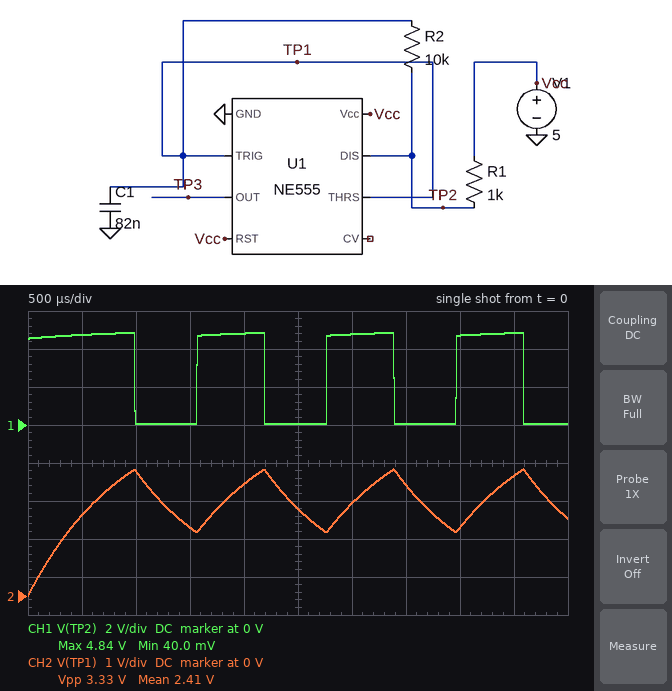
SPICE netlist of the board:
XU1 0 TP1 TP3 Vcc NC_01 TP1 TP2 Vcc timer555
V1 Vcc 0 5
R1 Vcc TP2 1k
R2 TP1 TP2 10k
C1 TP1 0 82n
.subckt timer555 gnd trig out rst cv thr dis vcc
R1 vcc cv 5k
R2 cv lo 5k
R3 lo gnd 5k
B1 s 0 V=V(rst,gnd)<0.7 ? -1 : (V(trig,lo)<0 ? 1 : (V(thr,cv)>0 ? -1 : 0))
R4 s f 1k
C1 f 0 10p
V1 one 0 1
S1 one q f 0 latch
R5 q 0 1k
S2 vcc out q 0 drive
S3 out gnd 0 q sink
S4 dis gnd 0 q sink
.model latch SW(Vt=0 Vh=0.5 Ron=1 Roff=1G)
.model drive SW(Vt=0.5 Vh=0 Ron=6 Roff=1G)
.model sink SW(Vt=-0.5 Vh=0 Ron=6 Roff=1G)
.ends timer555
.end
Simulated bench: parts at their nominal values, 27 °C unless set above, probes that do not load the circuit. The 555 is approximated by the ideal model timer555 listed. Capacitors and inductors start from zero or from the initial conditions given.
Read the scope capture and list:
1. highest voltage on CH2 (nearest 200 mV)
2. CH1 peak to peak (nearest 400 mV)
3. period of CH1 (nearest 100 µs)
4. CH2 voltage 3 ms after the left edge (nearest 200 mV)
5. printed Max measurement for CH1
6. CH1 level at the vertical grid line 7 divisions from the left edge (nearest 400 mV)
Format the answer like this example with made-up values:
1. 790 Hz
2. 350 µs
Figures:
1. 3.4 V
2. 4.8 V
3. 1.2 ms
4. 2.4 V
5. 4.84 V
6. 0 V
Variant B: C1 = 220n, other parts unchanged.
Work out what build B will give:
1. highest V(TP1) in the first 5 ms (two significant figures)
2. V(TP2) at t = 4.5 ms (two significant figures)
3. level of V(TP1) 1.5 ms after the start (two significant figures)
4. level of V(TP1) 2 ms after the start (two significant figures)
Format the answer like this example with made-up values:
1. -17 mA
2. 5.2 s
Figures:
1. 3.3 V
2. 4.7 V
3. 2.3 V
4. 2.8 V
